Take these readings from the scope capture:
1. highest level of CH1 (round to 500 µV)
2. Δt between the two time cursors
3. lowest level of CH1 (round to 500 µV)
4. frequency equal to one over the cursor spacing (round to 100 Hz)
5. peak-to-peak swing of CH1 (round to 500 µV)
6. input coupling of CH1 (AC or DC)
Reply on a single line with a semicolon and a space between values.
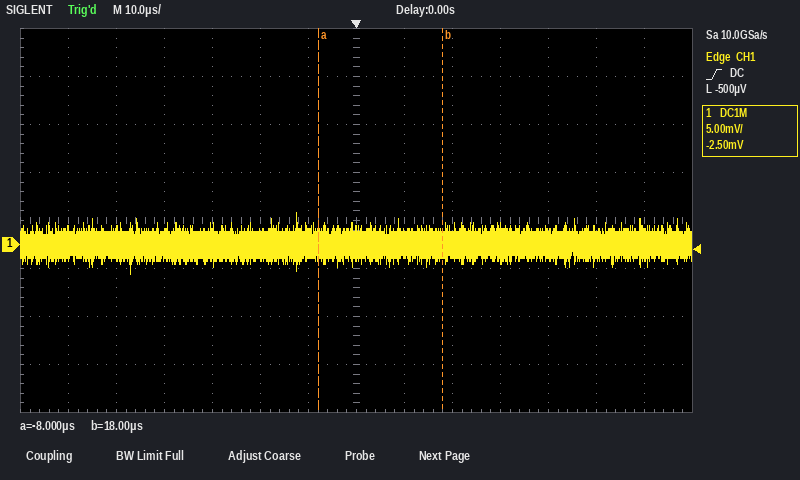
3.5 mV; 26 µs; -3.0 mV; 38.5 kHz; 6.5 mV; DC
